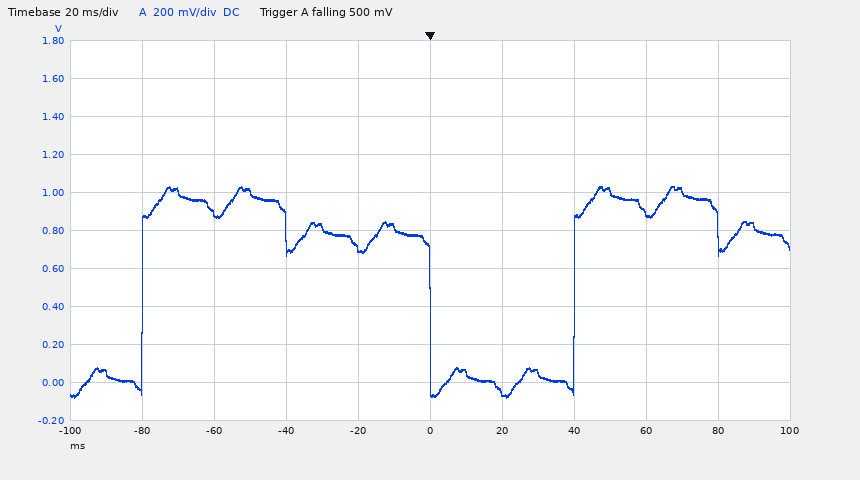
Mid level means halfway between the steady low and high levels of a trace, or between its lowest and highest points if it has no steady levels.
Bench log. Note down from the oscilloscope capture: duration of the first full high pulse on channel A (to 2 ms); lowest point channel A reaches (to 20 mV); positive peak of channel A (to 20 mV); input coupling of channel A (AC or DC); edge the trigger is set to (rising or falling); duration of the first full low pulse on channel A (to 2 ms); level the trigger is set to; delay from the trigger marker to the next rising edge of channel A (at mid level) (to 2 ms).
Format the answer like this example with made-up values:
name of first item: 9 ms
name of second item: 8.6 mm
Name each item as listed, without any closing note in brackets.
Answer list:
duration of the first full high pulse on channel A: 80 ms
lowest point channel A reaches: -80 mV
positive peak of channel A: 1.04 V
input coupling of channel A: DC
edge the trigger is set to: falling
duration of the first full low pulse on channel A: 40 ms
level the trigger is set to: 500 mV
delay from the trigger marker to the next rising edge of channel A (at mid level): 40 ms
